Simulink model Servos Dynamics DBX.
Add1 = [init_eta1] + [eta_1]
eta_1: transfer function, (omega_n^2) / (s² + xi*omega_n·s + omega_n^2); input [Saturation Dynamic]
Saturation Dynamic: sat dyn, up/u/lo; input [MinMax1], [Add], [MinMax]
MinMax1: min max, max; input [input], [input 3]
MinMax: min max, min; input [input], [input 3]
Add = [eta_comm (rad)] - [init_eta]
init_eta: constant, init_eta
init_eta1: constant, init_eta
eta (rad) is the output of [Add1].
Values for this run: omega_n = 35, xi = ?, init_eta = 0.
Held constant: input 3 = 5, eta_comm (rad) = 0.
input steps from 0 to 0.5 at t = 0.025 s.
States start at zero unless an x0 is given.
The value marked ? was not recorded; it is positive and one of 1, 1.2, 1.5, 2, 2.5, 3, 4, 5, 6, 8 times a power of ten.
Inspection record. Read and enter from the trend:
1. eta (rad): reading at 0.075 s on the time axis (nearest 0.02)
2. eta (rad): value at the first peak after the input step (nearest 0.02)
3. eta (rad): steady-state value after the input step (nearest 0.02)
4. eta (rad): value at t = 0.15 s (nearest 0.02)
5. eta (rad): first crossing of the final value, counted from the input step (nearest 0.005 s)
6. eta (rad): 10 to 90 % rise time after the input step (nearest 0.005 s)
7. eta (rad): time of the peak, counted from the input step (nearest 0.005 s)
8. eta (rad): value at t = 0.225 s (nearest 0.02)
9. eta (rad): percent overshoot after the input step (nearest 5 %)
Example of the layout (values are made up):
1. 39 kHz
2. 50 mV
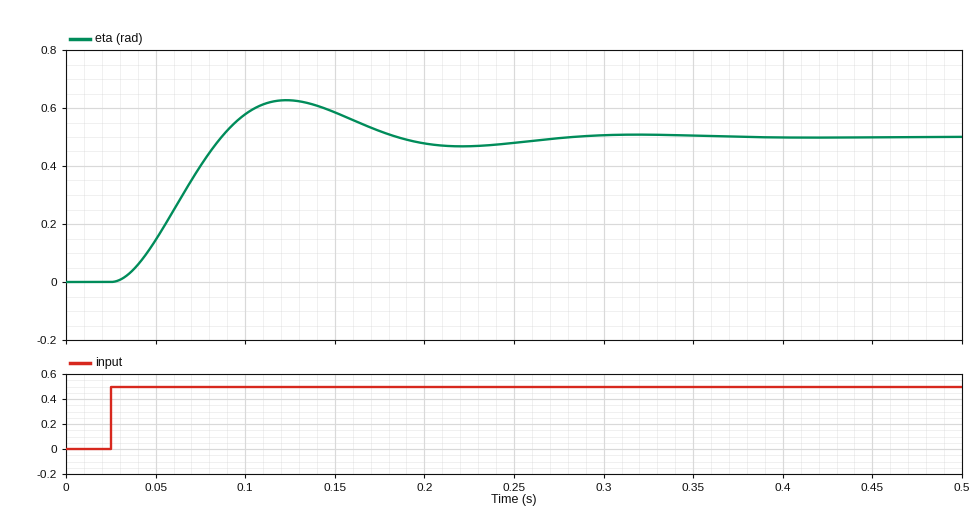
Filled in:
1. 0.40
2. 0.62
3. 0.50
4. 0.58
5. 0.060 s
6. 0.040 s
7. 0.100 s
8. 0.46
9. 25 %
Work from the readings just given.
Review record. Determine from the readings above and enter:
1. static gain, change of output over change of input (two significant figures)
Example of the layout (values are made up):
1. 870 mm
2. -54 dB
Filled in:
1. 1.0
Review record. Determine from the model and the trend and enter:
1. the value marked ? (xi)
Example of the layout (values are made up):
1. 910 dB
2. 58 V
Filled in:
1. 0.8
